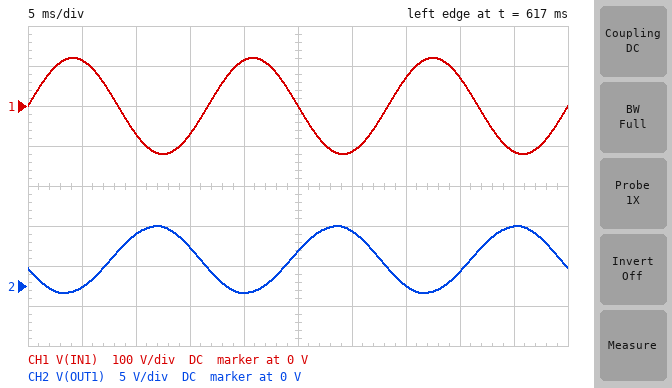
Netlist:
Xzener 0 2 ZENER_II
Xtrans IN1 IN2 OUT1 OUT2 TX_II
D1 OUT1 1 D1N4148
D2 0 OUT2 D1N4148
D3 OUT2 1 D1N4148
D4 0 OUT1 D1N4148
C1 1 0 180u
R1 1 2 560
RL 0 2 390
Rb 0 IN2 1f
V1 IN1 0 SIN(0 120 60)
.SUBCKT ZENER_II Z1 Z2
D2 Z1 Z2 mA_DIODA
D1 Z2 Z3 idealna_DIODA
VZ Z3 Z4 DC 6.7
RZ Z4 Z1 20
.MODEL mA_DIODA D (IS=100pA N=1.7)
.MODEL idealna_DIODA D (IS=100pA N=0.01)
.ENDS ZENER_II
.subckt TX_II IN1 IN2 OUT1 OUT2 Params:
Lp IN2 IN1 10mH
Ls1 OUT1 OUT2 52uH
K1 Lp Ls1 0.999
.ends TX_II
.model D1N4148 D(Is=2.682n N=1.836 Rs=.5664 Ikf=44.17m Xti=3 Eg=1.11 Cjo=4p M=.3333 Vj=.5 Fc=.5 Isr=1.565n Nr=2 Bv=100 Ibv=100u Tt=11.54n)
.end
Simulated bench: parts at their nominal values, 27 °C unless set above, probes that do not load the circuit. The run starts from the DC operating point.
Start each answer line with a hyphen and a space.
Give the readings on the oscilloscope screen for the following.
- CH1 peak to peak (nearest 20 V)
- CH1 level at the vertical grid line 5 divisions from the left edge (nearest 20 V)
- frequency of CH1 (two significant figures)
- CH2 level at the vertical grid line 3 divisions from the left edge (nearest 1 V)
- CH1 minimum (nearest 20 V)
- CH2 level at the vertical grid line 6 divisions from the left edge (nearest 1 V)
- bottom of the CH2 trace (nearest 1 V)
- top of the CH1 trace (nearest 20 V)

- 240 V
- 0 V
- 60 Hz
- 5 V
- -120 V
- 7 V
- -1 V
- 120 V
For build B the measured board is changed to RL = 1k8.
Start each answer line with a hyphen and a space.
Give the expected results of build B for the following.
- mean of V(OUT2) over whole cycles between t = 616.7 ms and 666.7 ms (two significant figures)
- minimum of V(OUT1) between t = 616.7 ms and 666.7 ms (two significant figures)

- 3.4 V
- -810 mV
